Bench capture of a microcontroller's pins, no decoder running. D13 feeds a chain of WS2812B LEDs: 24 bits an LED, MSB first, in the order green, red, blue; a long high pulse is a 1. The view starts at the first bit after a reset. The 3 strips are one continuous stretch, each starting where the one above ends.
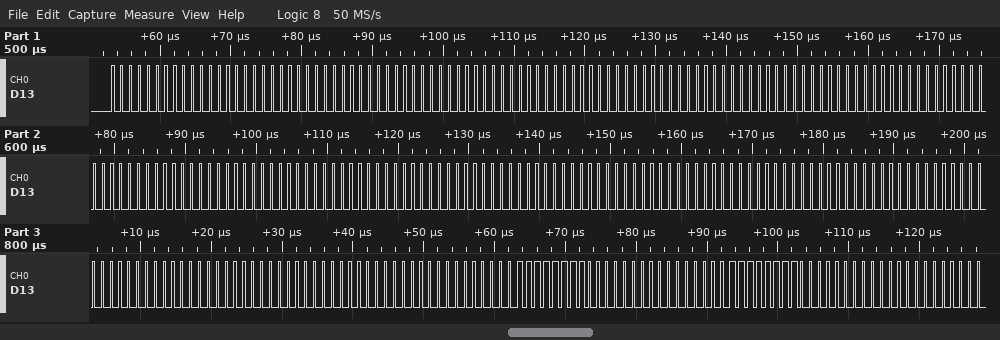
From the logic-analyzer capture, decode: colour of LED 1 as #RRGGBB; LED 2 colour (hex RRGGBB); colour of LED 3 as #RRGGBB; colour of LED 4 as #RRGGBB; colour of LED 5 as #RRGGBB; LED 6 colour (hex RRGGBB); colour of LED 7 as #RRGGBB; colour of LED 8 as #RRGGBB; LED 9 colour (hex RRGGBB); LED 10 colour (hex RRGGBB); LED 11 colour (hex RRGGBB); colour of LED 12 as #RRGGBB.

#000000
#000000
#000000
#000000
#000000
#000000
#000000
#000000
#000000
#000000
#FF0000
#FF0000
